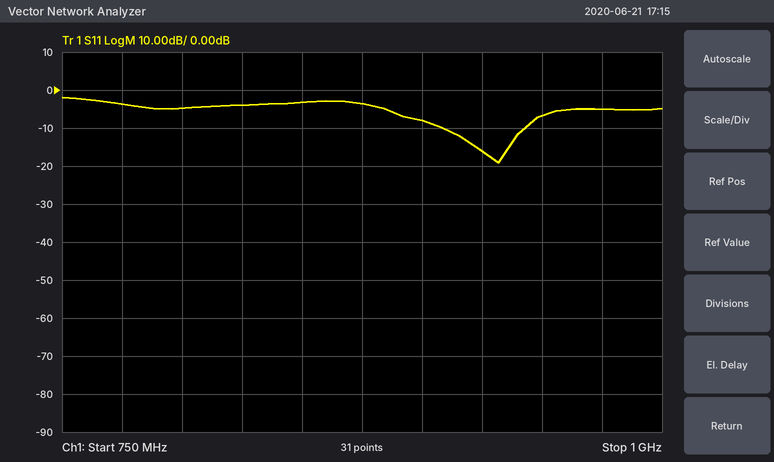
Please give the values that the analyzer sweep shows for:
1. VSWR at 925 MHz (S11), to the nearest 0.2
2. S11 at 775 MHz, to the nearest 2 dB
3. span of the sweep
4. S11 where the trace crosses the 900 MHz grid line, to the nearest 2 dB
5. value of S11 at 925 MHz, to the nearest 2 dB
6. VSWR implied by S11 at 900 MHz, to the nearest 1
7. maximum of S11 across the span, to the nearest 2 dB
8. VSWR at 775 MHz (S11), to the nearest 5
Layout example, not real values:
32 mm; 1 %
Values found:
1.4; -4 dB; 250 MHz; -8 dB; -16 dB; 2; -2 dB; 5
